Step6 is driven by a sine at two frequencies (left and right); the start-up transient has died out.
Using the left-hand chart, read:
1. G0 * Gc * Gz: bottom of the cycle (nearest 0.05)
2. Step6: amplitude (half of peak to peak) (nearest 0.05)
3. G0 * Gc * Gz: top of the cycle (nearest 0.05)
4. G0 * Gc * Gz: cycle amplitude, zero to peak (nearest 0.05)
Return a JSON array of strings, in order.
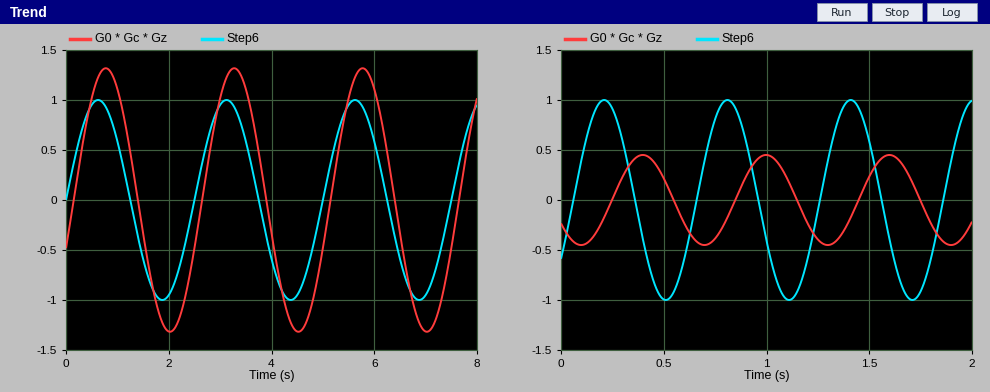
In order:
["-1.30", "1.00", "1.30", "1.30"]
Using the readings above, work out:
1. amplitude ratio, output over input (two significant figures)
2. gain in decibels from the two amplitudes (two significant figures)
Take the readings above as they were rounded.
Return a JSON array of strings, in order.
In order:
["1.3", "2.3 dB"]
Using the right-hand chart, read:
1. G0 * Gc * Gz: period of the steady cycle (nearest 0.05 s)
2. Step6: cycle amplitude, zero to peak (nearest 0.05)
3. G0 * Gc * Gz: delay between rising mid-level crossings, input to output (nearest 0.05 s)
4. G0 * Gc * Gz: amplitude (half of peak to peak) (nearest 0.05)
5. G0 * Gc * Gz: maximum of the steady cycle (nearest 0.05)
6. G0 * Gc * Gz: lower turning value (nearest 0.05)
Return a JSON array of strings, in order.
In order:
["0.60 s", "1.00", "0.20 s", "0.45", "0.45", "-0.45"]
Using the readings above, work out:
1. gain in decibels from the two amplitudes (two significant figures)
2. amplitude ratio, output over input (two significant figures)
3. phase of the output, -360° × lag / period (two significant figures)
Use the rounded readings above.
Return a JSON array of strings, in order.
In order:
["-6.9 dB", "0.45", "-120°"]
